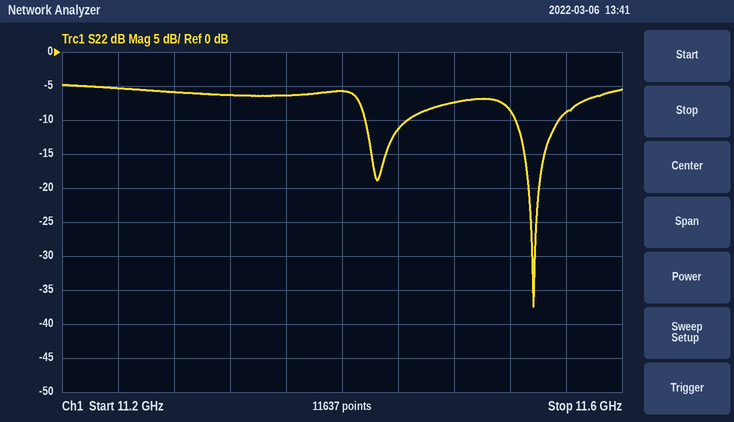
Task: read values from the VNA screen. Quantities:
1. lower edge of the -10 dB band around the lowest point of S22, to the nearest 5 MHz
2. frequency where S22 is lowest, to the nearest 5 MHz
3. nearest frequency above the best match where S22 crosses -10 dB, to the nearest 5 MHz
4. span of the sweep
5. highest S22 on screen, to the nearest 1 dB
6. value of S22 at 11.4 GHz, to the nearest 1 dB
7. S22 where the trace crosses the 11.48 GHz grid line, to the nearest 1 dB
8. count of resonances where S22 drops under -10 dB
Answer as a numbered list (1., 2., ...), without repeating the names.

1. 11.525 GHz
2. 11.535 GHz
3. 11.555 GHz
4. 400 MHz
5. -5 dB
6. -6 dB
7. -7 dB
8. 2
